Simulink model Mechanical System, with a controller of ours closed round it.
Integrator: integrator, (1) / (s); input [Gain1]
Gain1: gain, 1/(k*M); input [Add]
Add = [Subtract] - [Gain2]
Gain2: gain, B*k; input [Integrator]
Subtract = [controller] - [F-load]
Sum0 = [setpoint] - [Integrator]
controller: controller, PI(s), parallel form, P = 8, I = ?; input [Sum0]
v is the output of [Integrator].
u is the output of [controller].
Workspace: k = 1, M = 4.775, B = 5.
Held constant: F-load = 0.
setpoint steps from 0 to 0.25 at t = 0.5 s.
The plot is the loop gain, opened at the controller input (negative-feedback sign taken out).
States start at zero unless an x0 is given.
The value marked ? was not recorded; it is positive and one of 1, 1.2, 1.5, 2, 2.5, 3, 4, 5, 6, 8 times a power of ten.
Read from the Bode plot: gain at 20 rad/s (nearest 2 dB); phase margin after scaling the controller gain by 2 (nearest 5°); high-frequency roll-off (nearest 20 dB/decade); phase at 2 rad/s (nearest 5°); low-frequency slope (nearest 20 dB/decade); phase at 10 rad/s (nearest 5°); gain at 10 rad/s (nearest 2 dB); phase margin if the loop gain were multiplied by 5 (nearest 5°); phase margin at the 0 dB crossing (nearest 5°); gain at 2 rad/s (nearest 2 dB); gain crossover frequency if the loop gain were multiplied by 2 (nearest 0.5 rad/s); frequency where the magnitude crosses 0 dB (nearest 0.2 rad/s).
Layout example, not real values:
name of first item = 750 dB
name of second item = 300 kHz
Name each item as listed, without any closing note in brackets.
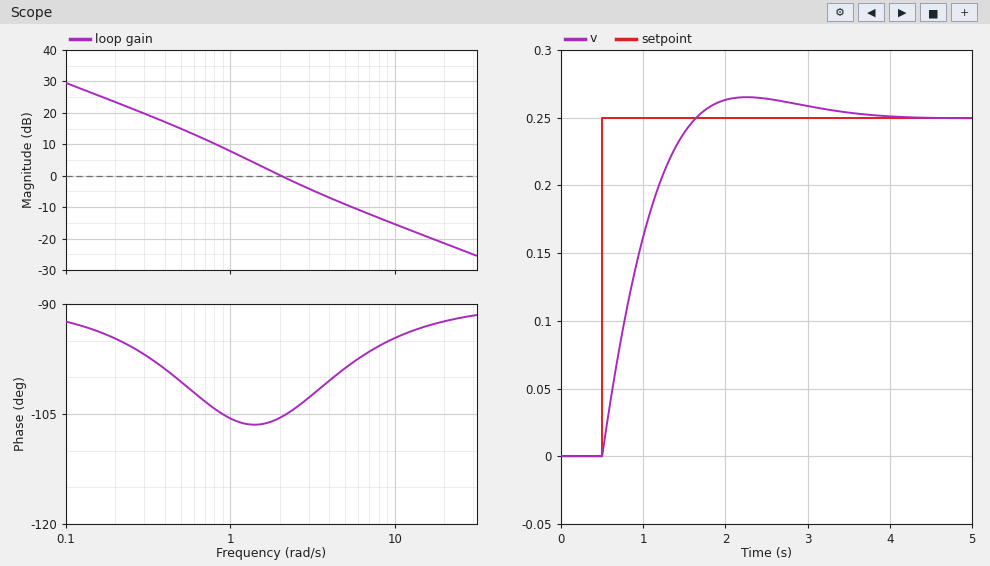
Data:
gain at 20 rad/s = -22 dB
phase margin after scaling the controller gain by 2 = 80°
high-frequency roll-off = -20 dB/decade
phase at 2 rad/s = -105°
low-frequency slope = -20 dB/decade
phase at 10 rad/s = -95°
gain at 10 rad/s = -16 dB
phase margin if the loop gain were multiplied by 5 = 85°
phase margin at the 0 dB crossing = 75°
gain at 2 rad/s = 0 dB
gain crossover frequency if the loop gain were multiplied by 2 = 3.5 rad/s
frequency where the magnitude crosses 0 dB = 2.0 rad/s
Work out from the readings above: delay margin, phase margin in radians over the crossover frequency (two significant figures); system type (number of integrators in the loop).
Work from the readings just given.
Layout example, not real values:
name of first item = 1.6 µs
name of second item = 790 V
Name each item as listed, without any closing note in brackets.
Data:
delay margin, phase margin in radians over the crossover frequency = 0.65 s
system type = 1
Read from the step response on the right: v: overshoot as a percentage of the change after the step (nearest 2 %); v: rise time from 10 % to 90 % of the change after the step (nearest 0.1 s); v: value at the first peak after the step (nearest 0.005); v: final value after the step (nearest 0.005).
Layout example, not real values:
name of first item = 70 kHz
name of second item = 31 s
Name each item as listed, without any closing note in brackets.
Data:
v: overshoot as a percentage of the change after the step = 6 %
v: rise time from 10 % to 90 % of the change after the step = 0.8 s
v: value at the first peak after the step = 0.265
v: final value after the step = 0.250
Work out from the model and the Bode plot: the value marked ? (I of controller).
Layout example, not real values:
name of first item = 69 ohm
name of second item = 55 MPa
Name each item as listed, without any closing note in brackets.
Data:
the value marked ? = 15
